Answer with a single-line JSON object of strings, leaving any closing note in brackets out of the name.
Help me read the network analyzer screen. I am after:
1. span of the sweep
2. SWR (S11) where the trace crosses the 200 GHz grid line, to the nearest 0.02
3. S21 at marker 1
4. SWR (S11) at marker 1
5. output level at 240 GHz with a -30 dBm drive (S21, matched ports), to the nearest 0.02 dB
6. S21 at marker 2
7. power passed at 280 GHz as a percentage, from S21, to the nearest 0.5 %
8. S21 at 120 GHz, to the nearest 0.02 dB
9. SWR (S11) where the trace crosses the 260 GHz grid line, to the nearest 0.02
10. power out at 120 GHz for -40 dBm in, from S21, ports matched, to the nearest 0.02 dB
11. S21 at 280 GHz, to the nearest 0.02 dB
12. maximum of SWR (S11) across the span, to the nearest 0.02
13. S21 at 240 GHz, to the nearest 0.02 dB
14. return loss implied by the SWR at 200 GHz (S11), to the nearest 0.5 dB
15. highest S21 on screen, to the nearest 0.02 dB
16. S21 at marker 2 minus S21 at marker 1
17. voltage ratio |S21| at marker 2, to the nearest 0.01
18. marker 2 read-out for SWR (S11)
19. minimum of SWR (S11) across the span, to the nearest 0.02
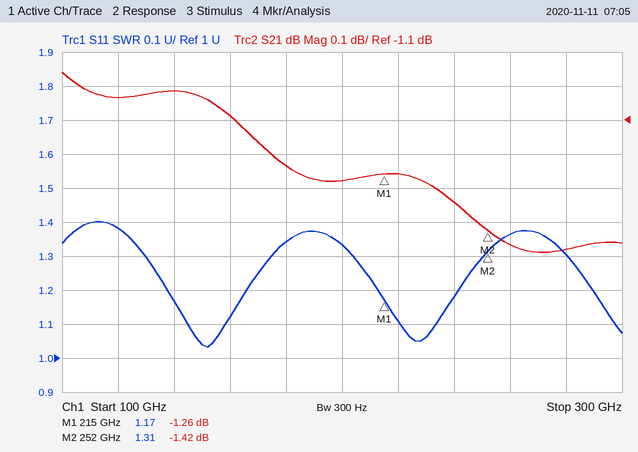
{"span of the sweep": "200 GHz", "SWR (S11) where the trace crosses the 200 GHz grid line, to the nearest 0.02": "1.34", "S21 at marker 1": "-1.26 dB", "SWR (S11) at marker 1": "1.17", "output level at 240 GHz with a -30 dBm drive (S21, matched ports), to the nearest 0.02 dB": "-31.34 dBm", "S21 at marker 2": "-1.42 dB", "power passed at 280 GHz as a percentage, from S21, to the nearest 0.5 %": "71.0 %", "S21 at 120 GHz, to the nearest 0.02 dB": "-1.04 dB", "SWR (S11) where the trace crosses the 260 GHz grid line, to the nearest 0.02": "1.36", "power out at 120 GHz for -40 dBm in, from S21, ports matched, to the nearest 0.02 dB": "-41.04 dBm", "S21 at 280 GHz, to the nearest 0.02 dB": "-1.48 dB", "maximum of SWR (S11) across the span, to the nearest 0.02": "1.40", "S21 at 240 GHz, to the nearest 0.02 dB": "-1.34 dB", "return loss implied by the SWR at 200 GHz (S11), to the nearest 0.5 dB": "17.0 dB", "highest S21 on screen, to the nearest 0.02 dB": "-0.96 dB", "S21 at marker 2 minus S21 at marker 1": "-0.16 dB", "voltage ratio |S21| at marker 2, to the nearest 0.01": "0.85", "marker 2 read-out for SWR": "1.31", "minimum of SWR (S11) across the span, to the nearest 0.02": "1.04"}
